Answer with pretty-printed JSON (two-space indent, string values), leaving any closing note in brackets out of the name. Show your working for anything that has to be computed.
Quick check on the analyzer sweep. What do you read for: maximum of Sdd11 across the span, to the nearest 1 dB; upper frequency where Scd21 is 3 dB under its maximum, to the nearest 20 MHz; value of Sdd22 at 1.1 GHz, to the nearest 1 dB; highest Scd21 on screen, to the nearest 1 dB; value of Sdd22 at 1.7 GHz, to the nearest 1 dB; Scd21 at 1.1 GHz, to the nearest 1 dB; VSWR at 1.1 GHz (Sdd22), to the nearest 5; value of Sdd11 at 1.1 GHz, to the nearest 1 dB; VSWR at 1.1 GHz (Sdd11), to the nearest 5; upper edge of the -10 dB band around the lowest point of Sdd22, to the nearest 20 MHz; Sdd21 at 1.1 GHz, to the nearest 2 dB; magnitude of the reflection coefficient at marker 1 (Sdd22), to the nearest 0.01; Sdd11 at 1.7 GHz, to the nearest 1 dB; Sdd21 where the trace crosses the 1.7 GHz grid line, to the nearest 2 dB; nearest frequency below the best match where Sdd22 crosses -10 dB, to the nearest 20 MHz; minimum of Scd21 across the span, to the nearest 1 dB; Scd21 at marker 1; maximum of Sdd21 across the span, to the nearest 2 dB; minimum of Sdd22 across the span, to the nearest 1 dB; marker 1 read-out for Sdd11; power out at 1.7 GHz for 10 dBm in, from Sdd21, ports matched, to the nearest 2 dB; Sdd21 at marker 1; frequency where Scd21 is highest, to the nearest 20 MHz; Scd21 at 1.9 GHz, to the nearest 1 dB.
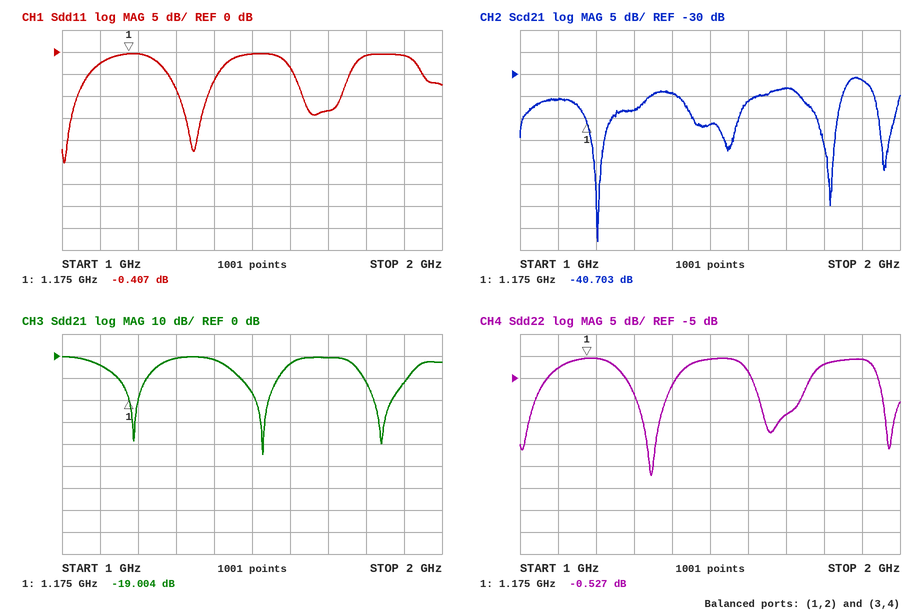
{
  "maximum of Sdd11 across the span, to the nearest 1 dB": "0 dB",
  "upper frequency where Scd21 is 3 dB under its maximum, to the nearest 20 MHz": "1.92 GHz",
  "value of Sdd22 at 1.1 GHz, to the nearest 1 dB": "-3 dB",
  "highest Scd21 on screen, to the nearest 1 dB": "-31 dB",
  "value of Sdd22 at 1.7 GHz, to the nearest 1 dB": "-13 dB",
  "Scd21 at 1.1 GHz, to the nearest 1 dB": "-36 dB",
  "VSWR at 1.1 GHz (Sdd22), to the nearest 5": "|Γ| = 10^(-3/20) = 0.7079; VSWR = (1 + 0.7079)/(1 − 0.7079) ≈ 5.85, so 5 to the nearest 5",
  "value of Sdd11 at 1.1 GHz, to the nearest 1 dB": "-3 dB",
  "VSWR at 1.1 GHz (Sdd11), to the nearest 5": "|Γ| = 10^(-3/20) = 0.7079; VSWR = (1 + 0.7079)/(1 − 0.7079) ≈ 5.85, so 5 to the nearest 5",
  "upper edge of the -10 dB band around the lowest point of Sdd22, to the nearest 20 MHz": "1.38 GHz",
  "Sdd21 at 1.1 GHz, to the nearest 2 dB": "-4 dB",
  "magnitude of the reflection coefficient at marker 1 (Sdd22), to the nearest 0.01": "10^(-0.527/20) ≈ 0.94",
  "Sdd11 at 1.7 GHz, to the nearest 1 dB": "-13 dB",
  "Sdd21 where the trace crosses the 1.7 GHz grid line, to the nearest 2 dB": "0 dB",
  "nearest frequency below the best match where Sdd22 crosses -10 dB, to the nearest 20 MHz": "1.30 GHz",
  "minimum of Scd21 across the span, to the nearest 1 dB": "-68 dB",
  "Scd21 at marker 1": "-40.703 dB",
  "maximum of Sdd21 across the span, to the nearest 2 dB": "0 dB",
  "minimum of Sdd22 across the span, to the nearest 1 dB": "-27 dB",
  "marker 1 read-out for Sdd11": "-0.407 dB",
  "power out at 1.7 GHz for 10 dBm in, from Sdd21, ports matched, to the nearest 2 dB": "10 dBm + (0 dB) = 10 dBm",
  "Sdd21 at marker 1": "-19.004 dB",
  "frequency where Scd21 is highest, to the nearest 20 MHz": "1.88 GHz",
  "Scd21 at 1.9 GHz, to the nearest 1 dB": "-31 dB"
}
